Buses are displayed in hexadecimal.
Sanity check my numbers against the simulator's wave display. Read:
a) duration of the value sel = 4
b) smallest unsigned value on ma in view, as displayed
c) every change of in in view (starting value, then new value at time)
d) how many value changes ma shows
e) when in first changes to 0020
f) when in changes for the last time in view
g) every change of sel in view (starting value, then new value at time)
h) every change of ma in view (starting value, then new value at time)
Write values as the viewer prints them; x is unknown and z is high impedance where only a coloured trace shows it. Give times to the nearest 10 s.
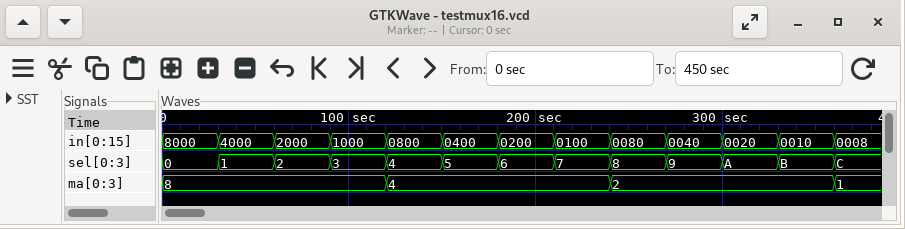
30 s
1
8000, 4000 at 30 s, 2000 at 60 s, 1000 at 90 s, 0800 at 120 s, 0400 at 150 s, 0200 at 180 s, 0100 at 210 s, 0080 at 240 s, 0040 at 270 s, 0020 at 300 s, 0010 at 330 s, 0008 at 360 s
3
300 s
360 s
0, 1 at 30 s, 2 at 60 s, 3 at 90 s, 4 at 120 s, 5 at 150 s, 6 at 180 s, 7 at 210 s, 8 at 240 s, 9 at 270 s, A at 300 s, B at 330 s, C at 360 s
8, 4 at 120 s, 2 at 240 s, 1 at 360 s
